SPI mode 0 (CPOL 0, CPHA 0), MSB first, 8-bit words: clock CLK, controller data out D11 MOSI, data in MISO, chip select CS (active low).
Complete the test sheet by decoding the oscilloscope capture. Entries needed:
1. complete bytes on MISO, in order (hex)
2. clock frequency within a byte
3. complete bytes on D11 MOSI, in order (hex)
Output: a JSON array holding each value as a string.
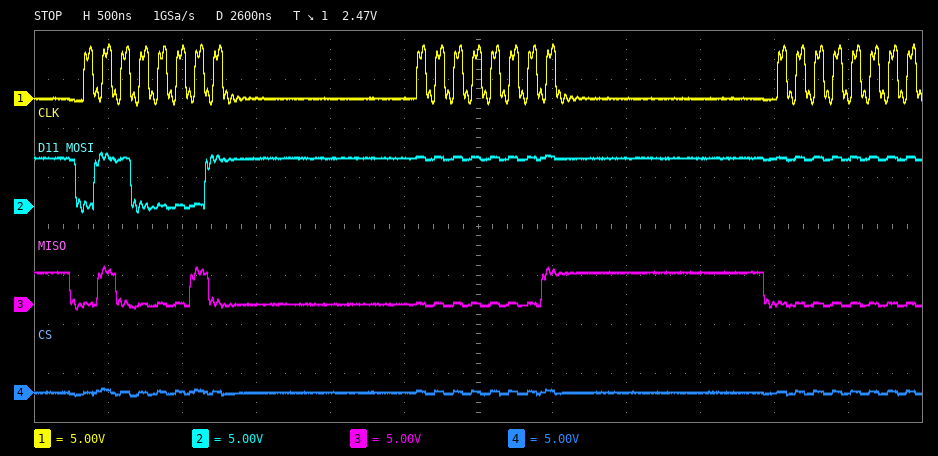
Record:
["42 01 00", "8 MHz", "61 FF FF"]
